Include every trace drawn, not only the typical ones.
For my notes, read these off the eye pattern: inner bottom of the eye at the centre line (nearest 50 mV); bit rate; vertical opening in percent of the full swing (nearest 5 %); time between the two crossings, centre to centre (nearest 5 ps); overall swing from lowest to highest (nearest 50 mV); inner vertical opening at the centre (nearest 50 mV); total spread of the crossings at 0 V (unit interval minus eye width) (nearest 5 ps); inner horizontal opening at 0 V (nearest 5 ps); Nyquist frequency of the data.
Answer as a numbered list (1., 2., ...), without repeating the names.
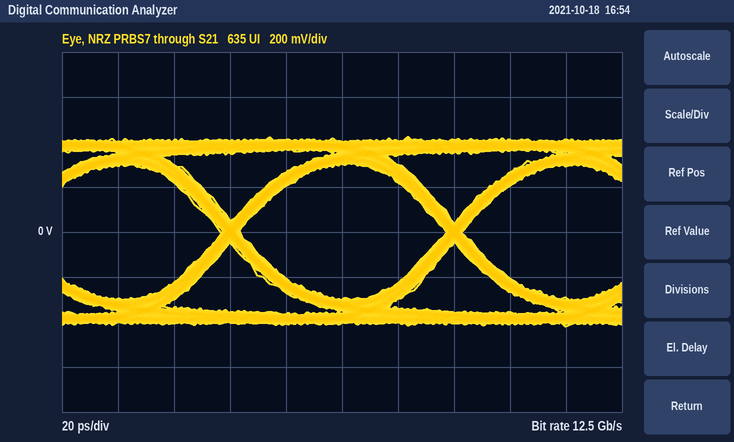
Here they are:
1. -300 mV
2. 12.5 Gb/s
3. 70 %
4. 80 ps
5. 850 mV
6. 600 mV
7. 5 ps
8. 75 ps
9. 6.25 GHz
